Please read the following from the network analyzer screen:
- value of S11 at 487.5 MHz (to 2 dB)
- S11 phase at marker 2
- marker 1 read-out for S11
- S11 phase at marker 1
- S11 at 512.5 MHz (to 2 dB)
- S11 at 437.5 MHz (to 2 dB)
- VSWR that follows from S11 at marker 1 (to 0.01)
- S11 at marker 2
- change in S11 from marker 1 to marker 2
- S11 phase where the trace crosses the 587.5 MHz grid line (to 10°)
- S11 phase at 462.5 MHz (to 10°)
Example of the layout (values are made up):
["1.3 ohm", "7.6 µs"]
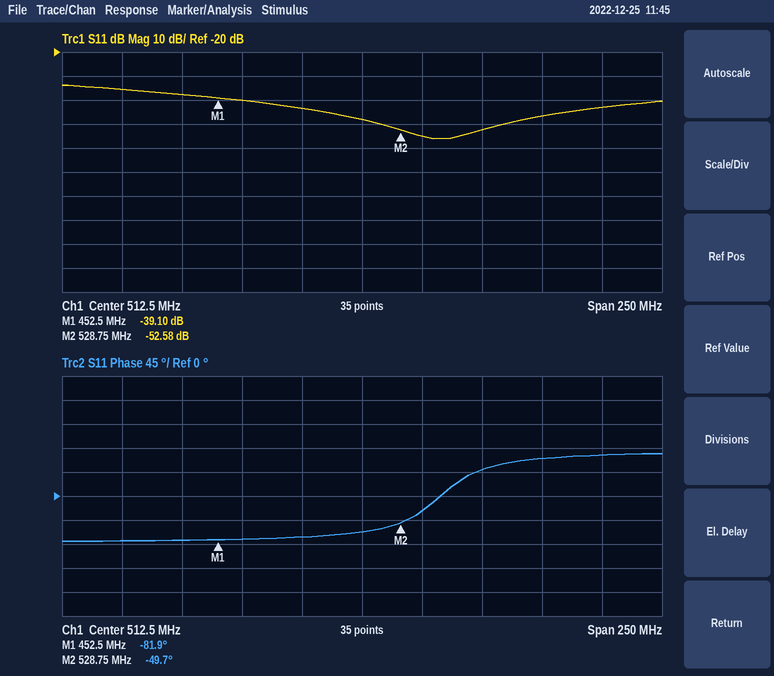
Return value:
["-44 dB", "-49.7°", "-39.10 dB", "-81.9°", "-48 dB", "-38 dB", "1.02", "-52.58 dB", "-13.48 dB", "70°", "-80°"]
